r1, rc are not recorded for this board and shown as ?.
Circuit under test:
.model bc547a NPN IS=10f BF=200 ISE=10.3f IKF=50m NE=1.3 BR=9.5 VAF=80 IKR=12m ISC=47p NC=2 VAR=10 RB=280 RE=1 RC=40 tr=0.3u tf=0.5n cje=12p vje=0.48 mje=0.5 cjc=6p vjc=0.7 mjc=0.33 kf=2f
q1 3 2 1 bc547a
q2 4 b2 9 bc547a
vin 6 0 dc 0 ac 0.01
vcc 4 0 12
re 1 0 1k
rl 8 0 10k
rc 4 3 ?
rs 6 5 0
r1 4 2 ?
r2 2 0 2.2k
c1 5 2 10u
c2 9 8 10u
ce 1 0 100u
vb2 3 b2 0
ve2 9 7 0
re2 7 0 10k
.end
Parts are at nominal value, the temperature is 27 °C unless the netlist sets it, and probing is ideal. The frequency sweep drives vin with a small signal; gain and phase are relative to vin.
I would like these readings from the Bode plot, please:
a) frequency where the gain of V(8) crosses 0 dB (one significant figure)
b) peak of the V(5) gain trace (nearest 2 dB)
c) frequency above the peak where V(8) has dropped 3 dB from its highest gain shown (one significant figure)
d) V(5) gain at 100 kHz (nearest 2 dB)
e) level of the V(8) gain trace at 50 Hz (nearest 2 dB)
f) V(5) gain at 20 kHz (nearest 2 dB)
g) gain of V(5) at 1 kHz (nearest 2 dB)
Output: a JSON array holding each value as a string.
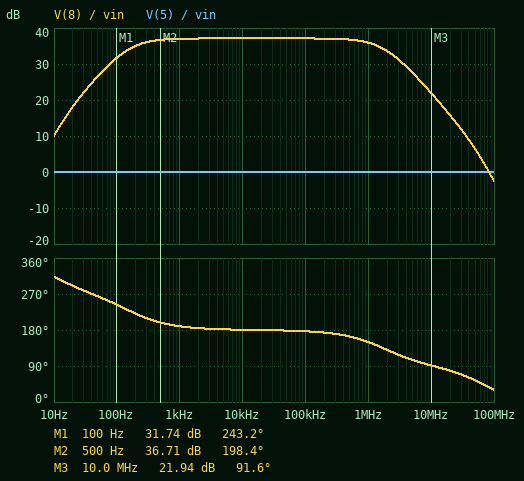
["80 MHz", "0 dB", "2 MHz", "0 dB", "26 dB", "0 dB", "0 dB"]
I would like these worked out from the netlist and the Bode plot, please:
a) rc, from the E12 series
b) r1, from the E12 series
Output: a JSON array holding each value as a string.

["820 Ω", "3.9 kΩ"]
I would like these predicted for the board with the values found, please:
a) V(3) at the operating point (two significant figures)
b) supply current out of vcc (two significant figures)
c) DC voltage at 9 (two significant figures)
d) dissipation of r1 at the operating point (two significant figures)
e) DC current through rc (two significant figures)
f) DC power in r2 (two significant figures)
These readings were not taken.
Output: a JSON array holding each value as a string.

["9.1 V", "6.4 mA", "8.4 V", "15 mW", "3.6 mA", "8.4 mW"]
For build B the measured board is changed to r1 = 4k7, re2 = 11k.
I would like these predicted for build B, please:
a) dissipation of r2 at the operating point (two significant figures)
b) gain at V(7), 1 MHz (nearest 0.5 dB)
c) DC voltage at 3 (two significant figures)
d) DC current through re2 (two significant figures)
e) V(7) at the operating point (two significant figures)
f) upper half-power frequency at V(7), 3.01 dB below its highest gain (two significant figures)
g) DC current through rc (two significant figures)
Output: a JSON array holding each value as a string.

["6.5 mW", "35.5 dB", "9.5 V", "800 µA", "8.8 V", "2.0 MHz", "3.1 mA"]
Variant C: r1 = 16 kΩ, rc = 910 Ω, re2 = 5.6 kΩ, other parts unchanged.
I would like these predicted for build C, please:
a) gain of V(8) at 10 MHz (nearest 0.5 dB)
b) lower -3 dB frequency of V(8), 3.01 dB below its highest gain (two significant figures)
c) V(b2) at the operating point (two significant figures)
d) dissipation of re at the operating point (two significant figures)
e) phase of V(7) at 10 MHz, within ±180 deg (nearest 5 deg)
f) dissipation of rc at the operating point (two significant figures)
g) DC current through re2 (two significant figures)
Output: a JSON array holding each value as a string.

["20.0 dB", "50 Hz", "11 V", "620 µW", "100 deg", "580 µW", "1.9 mA"]
